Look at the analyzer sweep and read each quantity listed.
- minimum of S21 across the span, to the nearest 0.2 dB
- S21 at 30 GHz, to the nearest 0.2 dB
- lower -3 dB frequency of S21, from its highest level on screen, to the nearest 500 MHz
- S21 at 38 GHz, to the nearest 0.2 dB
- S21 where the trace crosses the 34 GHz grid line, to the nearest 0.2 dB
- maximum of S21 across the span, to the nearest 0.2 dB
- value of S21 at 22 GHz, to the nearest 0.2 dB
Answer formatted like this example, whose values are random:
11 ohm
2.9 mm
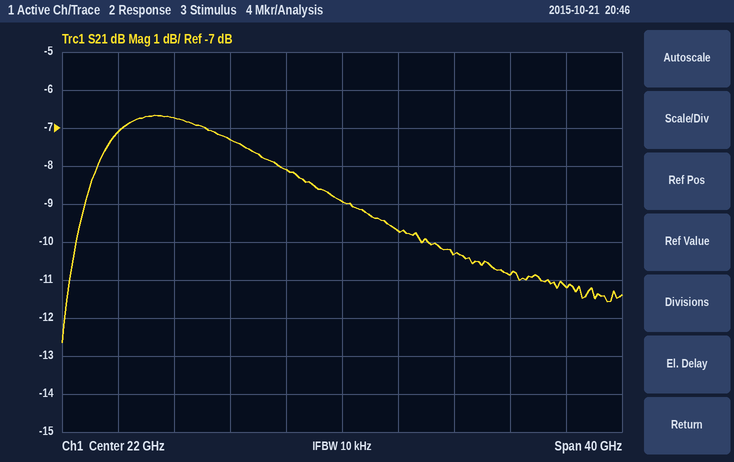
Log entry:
-12.6 dB
-10.4 dB
3.0 GHz
-11.2 dB
-10.8 dB
-6.6 dB
-9.0 dB
